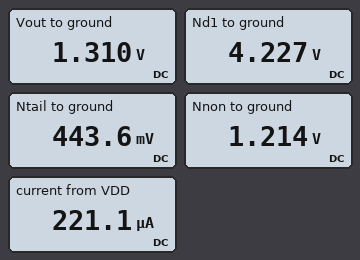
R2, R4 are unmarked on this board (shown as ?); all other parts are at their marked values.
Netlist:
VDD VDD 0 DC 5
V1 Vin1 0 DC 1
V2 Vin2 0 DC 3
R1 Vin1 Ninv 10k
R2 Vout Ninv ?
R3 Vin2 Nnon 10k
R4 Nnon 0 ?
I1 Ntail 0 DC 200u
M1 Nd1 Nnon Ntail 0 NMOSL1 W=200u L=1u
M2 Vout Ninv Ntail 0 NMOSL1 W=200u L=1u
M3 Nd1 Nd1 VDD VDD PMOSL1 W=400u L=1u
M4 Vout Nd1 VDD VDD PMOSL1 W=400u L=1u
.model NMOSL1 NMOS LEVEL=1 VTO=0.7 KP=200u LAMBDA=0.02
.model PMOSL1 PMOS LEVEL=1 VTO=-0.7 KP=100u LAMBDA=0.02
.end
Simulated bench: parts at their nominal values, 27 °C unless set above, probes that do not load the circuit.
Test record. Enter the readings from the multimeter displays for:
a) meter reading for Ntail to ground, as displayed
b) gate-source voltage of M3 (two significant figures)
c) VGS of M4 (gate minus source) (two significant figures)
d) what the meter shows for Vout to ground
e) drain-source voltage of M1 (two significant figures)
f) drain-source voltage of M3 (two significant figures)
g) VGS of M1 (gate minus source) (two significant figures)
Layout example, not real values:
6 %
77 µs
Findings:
443.6 mV
-770 mV
-770 mV
1.310 V
3.8 V
-770 mV
770 mV
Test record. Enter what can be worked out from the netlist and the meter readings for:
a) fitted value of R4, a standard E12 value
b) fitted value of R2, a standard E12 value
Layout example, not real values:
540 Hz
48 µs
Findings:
6.8 kΩ
4.7 kΩ
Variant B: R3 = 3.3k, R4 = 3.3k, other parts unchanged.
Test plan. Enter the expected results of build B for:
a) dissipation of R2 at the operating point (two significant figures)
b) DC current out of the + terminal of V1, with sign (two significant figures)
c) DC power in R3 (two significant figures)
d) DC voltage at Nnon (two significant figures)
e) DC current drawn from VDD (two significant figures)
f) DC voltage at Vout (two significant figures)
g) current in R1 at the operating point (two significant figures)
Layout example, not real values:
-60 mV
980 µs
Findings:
11 µW
-49 µA
680 µW
1.5 V
250 µA
1.7 V
49 µA
